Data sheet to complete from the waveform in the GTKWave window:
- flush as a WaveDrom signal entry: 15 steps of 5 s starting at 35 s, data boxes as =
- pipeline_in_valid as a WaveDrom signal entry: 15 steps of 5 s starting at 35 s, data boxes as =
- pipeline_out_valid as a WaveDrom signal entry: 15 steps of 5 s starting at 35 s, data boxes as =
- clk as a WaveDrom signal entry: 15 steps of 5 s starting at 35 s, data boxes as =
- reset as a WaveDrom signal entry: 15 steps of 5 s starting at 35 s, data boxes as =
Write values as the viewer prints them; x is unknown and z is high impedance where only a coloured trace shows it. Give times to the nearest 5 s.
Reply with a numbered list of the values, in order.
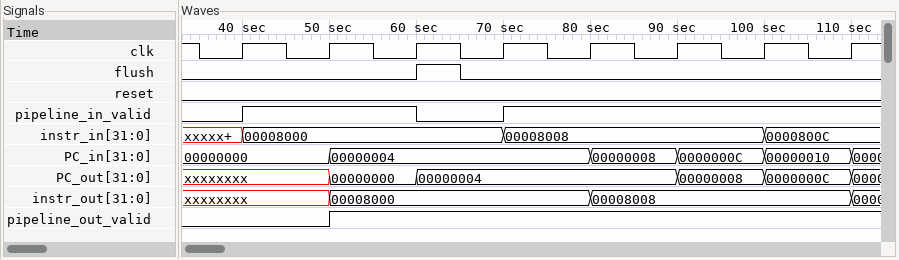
1. {name: 'flush', wave: '0....10........'}
2. {name: 'pipeline_in_valid', wave: '01...0.1.......'}
3. {name: 'pipeline_out_valid', wave: '0..1...........'}
4. {name: 'clk', wave: '010101010101010'}
5. {name: 'reset', wave: '0..............'}
